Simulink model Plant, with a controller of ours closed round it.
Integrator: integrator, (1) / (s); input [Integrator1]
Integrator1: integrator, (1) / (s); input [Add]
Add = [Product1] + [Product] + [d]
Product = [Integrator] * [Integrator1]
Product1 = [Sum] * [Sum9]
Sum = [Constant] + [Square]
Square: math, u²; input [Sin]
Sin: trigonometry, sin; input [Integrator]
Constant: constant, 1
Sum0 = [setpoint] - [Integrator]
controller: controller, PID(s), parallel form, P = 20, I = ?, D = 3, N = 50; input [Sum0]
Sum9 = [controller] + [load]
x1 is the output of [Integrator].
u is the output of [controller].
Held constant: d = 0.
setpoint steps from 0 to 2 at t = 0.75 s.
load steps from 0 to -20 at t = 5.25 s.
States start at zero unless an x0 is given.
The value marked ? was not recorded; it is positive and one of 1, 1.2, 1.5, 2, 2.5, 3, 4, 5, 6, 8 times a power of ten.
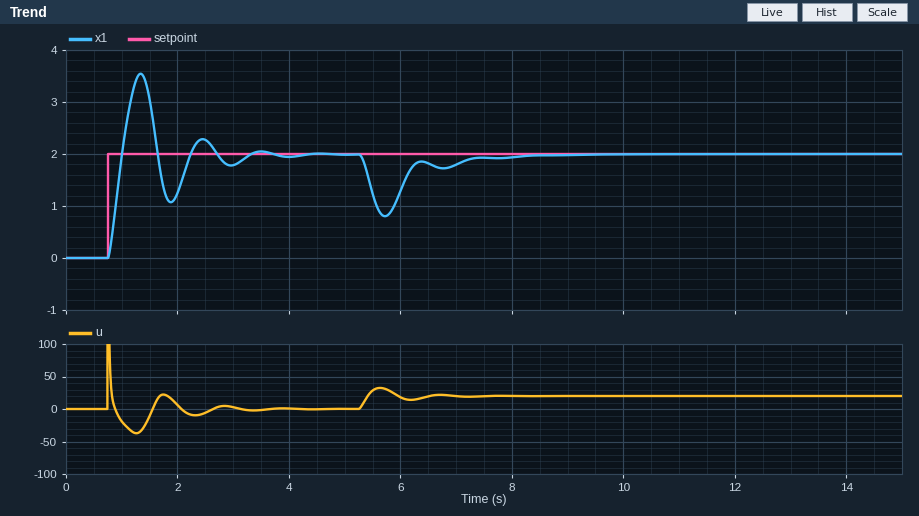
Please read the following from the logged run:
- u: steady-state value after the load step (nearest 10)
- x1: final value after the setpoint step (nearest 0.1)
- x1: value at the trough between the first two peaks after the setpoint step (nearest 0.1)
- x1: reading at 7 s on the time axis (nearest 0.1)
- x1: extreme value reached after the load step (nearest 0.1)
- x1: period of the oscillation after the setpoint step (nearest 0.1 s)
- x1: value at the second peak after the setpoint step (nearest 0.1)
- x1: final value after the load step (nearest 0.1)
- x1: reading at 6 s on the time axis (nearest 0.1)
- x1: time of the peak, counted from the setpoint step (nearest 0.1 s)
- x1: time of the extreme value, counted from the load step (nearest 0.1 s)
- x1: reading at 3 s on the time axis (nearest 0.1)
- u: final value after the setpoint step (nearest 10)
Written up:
20
2.0
1.1
1.8
0.8
1.1 s
2.3
2.0
1.3
0.6 s
0.5 s
1.8
0
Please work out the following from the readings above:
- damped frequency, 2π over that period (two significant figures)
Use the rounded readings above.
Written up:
5.7 rad/s
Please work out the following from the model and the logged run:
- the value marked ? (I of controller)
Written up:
20
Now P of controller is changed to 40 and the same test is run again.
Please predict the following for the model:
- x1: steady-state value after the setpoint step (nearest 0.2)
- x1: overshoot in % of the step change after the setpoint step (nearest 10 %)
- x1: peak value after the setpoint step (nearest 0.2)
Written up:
2.0
80 %
3.6
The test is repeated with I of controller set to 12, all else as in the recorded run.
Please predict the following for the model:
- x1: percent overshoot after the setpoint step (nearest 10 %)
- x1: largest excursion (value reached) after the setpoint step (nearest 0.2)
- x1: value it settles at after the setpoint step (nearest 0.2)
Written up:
70 %
3.4
2.0
